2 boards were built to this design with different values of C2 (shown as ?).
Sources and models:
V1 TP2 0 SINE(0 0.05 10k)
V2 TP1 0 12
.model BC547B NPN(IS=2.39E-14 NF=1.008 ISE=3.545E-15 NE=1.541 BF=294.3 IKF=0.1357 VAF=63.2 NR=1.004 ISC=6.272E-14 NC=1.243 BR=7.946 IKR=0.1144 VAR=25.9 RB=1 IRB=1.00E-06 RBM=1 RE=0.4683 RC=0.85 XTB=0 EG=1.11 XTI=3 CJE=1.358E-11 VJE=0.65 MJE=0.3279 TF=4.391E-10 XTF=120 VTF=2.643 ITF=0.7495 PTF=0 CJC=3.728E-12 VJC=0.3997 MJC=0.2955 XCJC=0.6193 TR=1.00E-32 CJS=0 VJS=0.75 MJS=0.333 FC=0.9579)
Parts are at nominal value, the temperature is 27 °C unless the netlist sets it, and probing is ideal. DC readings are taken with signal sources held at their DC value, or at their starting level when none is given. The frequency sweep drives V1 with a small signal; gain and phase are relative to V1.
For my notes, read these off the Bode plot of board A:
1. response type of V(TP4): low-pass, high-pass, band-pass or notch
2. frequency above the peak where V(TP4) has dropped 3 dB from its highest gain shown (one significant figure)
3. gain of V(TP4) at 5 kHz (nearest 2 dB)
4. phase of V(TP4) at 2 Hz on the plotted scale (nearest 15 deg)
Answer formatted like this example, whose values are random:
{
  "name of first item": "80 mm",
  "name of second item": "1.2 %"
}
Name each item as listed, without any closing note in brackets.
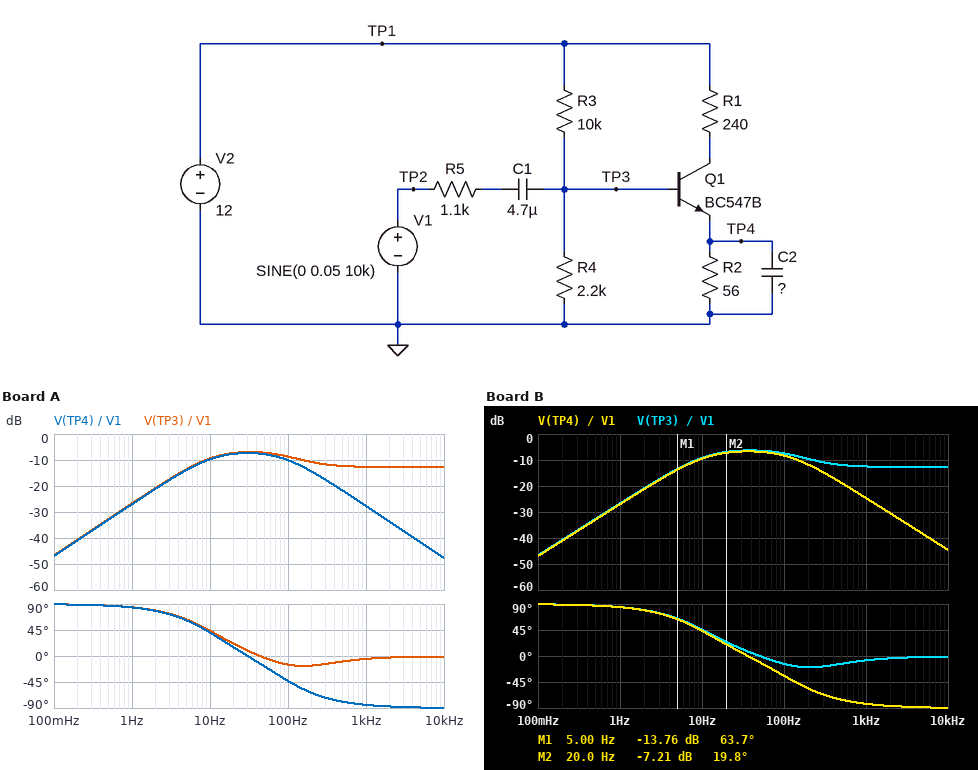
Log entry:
{
  "response type of V(TP4): low-pass, high-pass, band-pass or notch": "band-pass",
  "frequency above the peak where V(TP4) has dropped 3 dB from its highest gain shown": "100 Hz",
  "gain of V(TP4) at 5 kHz": "-42 dB",
  "phase of V(TP4) at 2 Hz on the plotted scale": "75 deg"
}
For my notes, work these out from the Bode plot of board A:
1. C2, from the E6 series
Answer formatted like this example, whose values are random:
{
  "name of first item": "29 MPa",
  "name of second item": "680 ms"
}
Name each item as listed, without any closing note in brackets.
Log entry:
{
  "C2, from the E6 series": "470 µF"
}
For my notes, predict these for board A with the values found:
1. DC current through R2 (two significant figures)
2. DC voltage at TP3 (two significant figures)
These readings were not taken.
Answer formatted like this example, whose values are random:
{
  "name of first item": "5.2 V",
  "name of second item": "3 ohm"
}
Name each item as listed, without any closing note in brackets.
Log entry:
{
  "DC current through R2": "23 mA",
  "DC voltage at TP3": "2.0 V"
}
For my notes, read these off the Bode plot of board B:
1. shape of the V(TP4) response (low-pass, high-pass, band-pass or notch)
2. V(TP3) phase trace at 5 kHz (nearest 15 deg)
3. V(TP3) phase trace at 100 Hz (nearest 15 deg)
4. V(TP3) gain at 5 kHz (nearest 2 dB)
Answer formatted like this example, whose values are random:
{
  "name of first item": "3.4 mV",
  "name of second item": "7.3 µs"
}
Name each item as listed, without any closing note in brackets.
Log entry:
{
  "shape of the V(TP4) response": "band-pass",
  "V(TP3) phase trace at 5 kHz": "0 deg",
  "V(TP3) phase trace at 100 Hz": "-15 deg",
  "V(TP3) gain at 5 kHz": "-12 dB"
}
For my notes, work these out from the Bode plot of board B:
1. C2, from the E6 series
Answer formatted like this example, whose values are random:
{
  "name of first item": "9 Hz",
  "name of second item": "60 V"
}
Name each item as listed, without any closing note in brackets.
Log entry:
{
  "C2, from the E6 series": "330 µF"
}
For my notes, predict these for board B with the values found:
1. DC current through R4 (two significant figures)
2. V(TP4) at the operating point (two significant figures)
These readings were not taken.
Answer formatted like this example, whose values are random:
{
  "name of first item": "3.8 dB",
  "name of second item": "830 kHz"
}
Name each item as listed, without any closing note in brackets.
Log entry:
{
  "DC current through R4": "910 µA",
  "V(TP4) at the operating point": "1.3 V"
}
